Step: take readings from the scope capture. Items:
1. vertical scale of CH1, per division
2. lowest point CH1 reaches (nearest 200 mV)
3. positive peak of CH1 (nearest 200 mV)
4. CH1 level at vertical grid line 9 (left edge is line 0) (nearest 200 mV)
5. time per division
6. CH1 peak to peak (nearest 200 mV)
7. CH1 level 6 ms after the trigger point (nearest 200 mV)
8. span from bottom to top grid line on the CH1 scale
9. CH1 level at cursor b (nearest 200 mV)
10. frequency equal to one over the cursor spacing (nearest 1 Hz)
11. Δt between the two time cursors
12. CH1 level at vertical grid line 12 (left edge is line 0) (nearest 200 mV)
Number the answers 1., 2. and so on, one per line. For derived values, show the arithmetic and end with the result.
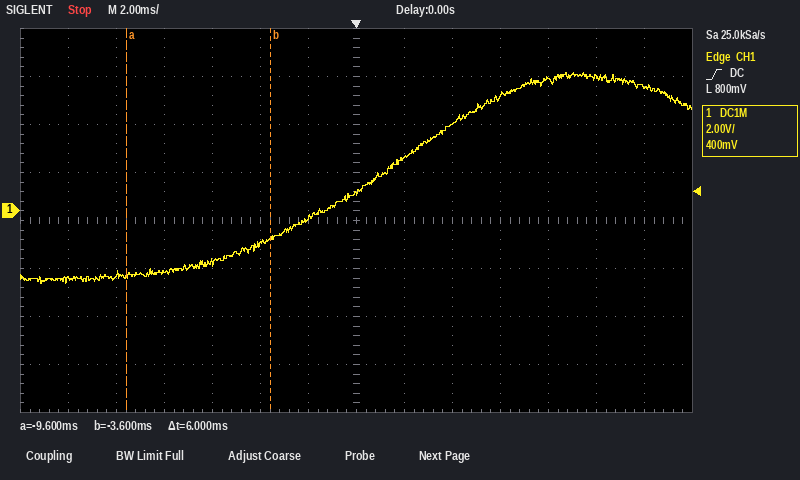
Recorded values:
1. 2 V
2. -3.0 V
3. 5.8 V
4. 3.6 V
5. 2 ms
6. 5.8 V − (-3.0 V) = 8.8 V
7. 4.8 V
8. 16 V
9. -1.2 V
10. 1 / 6 ms ≈ 167 Hz
11. 6 ms
12. 5.6 V
